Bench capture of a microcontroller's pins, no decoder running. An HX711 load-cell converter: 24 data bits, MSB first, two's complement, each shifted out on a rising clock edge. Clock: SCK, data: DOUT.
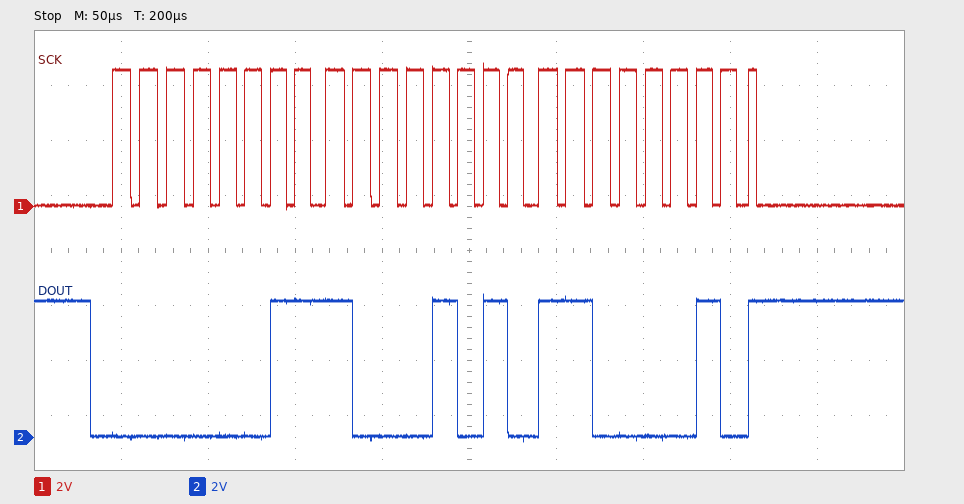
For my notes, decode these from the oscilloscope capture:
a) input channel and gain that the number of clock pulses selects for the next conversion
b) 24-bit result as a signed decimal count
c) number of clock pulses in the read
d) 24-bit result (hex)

channel A, gain 128
232130
25
0x038AC2
